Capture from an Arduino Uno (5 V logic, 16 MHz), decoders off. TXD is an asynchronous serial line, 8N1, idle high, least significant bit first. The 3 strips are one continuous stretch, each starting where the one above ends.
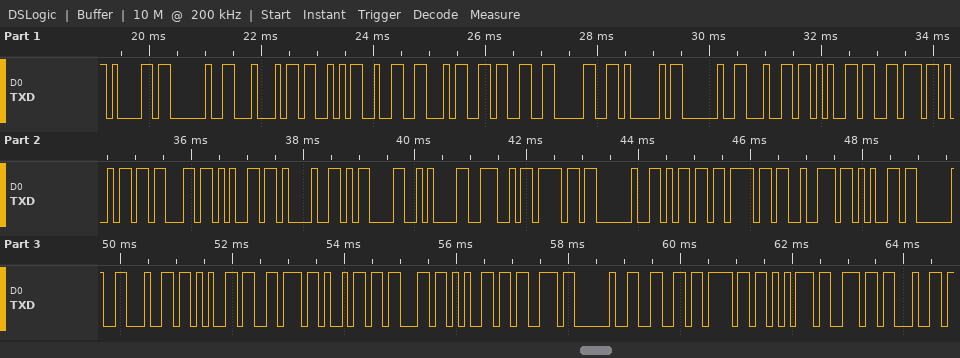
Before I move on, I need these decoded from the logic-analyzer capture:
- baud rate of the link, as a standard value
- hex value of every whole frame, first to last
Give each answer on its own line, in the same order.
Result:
9600 baud
0x61 0x20 0x44 0x53 0x32 0x34 0x33 0x30 0x41 0x20 0x64 0x65 0x76 0x69 0x63 0x65 0x21 0x0D 0x0A 0x4E 0x6F 0x20 0x6D 0x6F 0x72 0x65 0x20 0x64 0x65 0x76 0x69 0x63 0x65 0x73 0x20 0x66 0x6F 0x75 0x6E 0x64
